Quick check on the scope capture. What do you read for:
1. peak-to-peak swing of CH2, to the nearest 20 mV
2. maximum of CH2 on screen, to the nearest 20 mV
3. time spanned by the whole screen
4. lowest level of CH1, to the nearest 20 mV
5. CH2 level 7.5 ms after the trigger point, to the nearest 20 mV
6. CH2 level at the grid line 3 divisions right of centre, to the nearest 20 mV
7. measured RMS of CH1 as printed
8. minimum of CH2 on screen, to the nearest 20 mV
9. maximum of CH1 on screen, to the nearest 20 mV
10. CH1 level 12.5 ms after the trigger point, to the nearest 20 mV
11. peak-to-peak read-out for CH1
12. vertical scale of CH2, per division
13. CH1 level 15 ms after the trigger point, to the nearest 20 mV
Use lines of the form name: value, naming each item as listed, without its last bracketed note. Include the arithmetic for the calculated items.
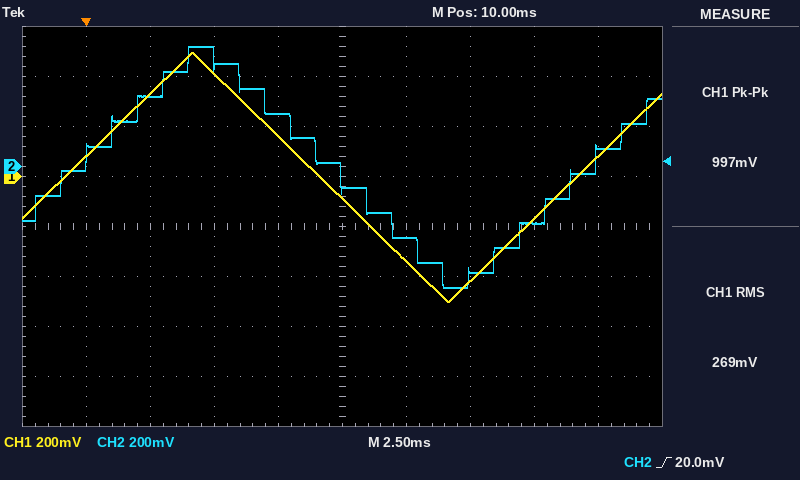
peak-to-peak swing of CH2, to the nearest 20 mV: 480 mV − (-480 mV) = 960 mV
maximum of CH2 on screen, to the nearest 20 mV: 480 mV
time spanned by the whole screen: 25 ms
lowest level of CH1, to the nearest 20 mV: -500 mV
CH2 level 7.5 ms after the trigger point, to the nearest 20 mV: 220 mV
CH2 level at the grid line 3 divisions right of centre, to the nearest 20 mV: -220 mV
measured RMS of CH1 as printed: 269 mV
minimum of CH2 on screen, to the nearest 20 mV: -480 mV
maximum of CH1 on screen, to the nearest 20 mV: 500 mV
CH1 level 12.5 ms after the trigger point, to the nearest 20 mV: -340 mV
peak-to-peak read-out for CH1: 997 mV
vertical scale of CH2, per division: 200 mV
CH1 level 15 ms after the trigger point, to the nearest 20 mV: -420 mV
